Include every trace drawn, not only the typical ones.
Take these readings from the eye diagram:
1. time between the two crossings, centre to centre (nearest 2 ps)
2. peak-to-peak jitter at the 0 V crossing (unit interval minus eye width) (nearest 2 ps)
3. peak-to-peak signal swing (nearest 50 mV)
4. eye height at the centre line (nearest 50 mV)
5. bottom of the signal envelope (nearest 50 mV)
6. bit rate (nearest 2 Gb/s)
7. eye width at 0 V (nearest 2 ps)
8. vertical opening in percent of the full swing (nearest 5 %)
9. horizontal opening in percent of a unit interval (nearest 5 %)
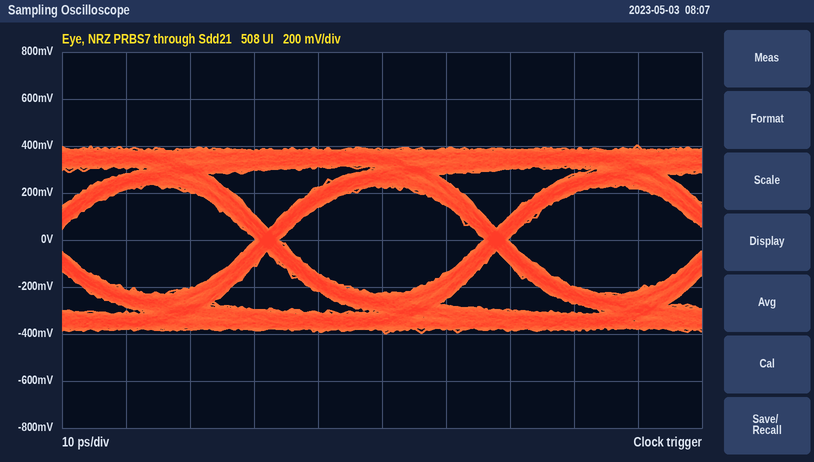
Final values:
36 ps
4 ps
800 mV
450 mV
-400 mV
28 Gb/s
32 ps
55 %
90 %
